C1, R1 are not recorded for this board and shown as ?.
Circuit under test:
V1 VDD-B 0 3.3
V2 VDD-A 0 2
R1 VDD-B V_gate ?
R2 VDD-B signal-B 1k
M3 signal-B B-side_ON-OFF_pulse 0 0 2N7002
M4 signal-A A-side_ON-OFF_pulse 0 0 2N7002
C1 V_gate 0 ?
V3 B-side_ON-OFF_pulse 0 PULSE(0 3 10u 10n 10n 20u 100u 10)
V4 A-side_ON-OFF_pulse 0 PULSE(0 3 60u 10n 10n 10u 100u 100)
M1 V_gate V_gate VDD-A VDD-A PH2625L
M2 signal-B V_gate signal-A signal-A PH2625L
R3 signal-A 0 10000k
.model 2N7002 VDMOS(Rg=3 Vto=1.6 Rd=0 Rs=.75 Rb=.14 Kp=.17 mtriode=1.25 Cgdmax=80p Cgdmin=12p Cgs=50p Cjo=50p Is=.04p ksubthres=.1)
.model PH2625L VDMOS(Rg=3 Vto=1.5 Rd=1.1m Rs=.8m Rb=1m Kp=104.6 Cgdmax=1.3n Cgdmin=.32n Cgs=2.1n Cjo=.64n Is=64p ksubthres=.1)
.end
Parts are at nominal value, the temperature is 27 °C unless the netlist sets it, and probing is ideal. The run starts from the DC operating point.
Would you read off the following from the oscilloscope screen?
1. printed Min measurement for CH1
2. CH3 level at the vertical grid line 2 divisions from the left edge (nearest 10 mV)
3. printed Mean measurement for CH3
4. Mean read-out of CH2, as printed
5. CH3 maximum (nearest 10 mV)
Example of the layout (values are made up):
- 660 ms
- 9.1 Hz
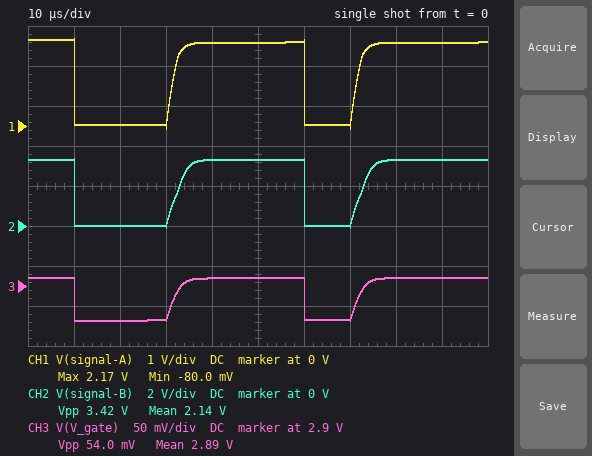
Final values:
- -80.0 mV
- 2.86 V
- 2.89 V
- 2.14 V
- 2.91 V
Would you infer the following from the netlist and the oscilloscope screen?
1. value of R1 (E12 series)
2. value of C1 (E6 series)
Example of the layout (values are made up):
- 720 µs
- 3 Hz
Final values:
- 100 kΩ
- 150 nF
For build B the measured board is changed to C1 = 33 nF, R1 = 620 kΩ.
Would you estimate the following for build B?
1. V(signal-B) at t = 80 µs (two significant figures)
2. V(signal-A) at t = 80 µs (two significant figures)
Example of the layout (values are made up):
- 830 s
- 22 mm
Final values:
- 3.3 V
- 2.0 V
